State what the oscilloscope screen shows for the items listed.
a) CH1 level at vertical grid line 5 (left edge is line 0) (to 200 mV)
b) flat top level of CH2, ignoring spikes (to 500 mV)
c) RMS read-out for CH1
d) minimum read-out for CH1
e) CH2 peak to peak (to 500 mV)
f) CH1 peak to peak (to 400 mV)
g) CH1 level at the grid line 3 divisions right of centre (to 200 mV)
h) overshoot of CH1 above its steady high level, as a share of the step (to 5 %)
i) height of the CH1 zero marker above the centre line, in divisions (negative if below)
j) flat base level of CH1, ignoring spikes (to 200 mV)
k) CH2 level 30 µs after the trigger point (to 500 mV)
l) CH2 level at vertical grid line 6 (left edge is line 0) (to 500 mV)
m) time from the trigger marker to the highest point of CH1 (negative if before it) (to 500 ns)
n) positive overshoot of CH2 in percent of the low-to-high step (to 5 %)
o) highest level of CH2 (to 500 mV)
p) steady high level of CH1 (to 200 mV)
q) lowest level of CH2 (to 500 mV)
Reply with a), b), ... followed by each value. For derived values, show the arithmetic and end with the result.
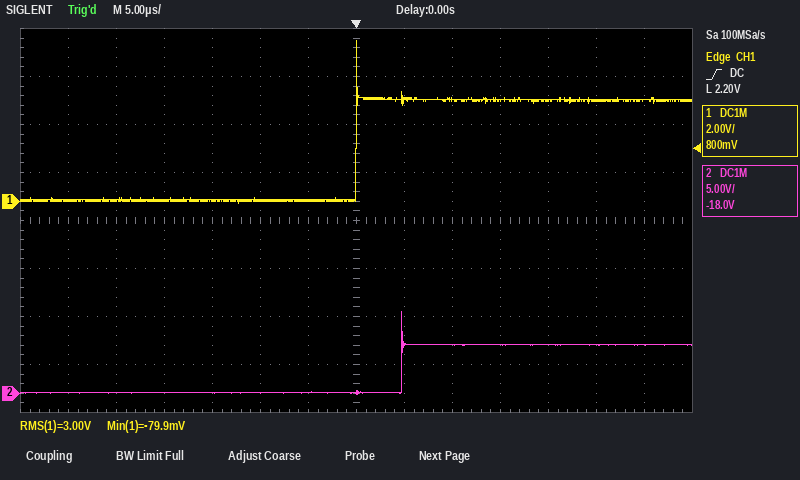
a) 0.0 V
b) 5.0 V
c) 3.00 V
d) -79.9 mV
e) 8.5 V − (0.0 V) = 8.5 V
f) 6.8 V
g) 4.2 V
h) 60 %
i) +0.4 div
j) 0.0 V
k) 5.0 V
l) 0.0 V
m) 0.0 µs
n) 70 %
o) 8.5 V
p) 4.2 V
q) 0.0 V
